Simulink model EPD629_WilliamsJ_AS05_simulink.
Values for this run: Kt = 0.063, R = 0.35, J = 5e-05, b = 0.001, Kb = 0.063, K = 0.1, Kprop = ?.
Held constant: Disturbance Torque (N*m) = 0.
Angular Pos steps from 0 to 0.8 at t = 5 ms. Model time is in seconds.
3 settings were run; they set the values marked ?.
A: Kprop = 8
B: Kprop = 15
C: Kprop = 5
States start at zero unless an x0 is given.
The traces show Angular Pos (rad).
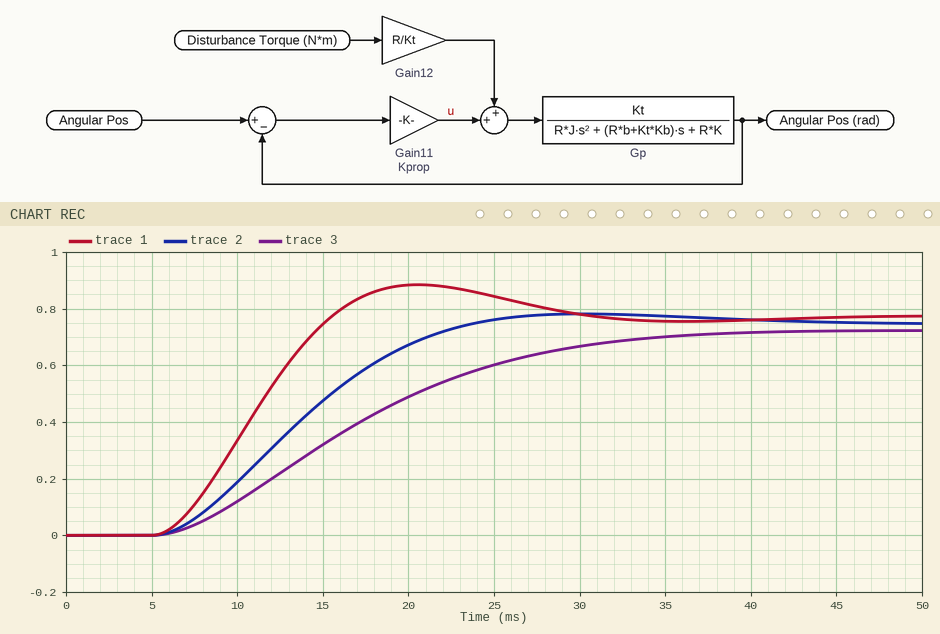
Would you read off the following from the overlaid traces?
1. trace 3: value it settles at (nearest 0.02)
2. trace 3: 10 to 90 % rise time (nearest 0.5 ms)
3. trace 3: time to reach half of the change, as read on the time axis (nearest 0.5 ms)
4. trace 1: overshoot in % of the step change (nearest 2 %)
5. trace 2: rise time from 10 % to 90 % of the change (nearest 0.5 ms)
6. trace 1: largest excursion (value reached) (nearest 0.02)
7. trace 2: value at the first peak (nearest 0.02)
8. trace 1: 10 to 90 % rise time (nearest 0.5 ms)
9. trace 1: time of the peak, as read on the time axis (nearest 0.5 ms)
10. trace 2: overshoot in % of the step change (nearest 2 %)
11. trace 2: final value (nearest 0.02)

0.72
19.5 ms
16.0 ms
14 %
12.0 ms
0.88
0.78
7.0 ms
20.5 ms
4 %
0.74
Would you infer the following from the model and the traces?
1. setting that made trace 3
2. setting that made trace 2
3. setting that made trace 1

C
A
B
